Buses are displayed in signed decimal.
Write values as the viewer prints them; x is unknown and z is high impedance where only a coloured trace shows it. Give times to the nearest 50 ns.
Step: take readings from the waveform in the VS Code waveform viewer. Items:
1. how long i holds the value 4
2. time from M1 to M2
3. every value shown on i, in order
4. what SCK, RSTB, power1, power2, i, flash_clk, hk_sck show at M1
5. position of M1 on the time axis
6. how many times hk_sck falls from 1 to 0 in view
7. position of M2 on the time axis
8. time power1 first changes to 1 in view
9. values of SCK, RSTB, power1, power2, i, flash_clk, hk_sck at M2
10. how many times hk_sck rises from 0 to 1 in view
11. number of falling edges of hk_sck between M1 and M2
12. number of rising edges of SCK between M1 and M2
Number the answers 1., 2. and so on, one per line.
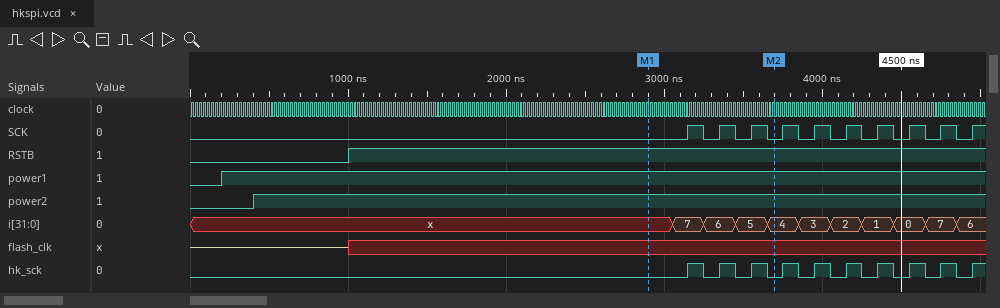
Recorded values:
1. 200 ns
2. 800 ns
3. x, 7, 6, 5, 4, 3, 2, 1, 0, 7, 6
4. SCK=0, RSTB=1, power1=1, power2=1, i=x, flash_clk=x, hk_sck=0
5. 2900 ns
6. 9
7. 3700 ns
8. 200 ns
9. SCK=0, RSTB=1, power1=1, power2=1, i=4, flash_clk=x, hk_sck=0
10. 10
11. 3
12. 3
